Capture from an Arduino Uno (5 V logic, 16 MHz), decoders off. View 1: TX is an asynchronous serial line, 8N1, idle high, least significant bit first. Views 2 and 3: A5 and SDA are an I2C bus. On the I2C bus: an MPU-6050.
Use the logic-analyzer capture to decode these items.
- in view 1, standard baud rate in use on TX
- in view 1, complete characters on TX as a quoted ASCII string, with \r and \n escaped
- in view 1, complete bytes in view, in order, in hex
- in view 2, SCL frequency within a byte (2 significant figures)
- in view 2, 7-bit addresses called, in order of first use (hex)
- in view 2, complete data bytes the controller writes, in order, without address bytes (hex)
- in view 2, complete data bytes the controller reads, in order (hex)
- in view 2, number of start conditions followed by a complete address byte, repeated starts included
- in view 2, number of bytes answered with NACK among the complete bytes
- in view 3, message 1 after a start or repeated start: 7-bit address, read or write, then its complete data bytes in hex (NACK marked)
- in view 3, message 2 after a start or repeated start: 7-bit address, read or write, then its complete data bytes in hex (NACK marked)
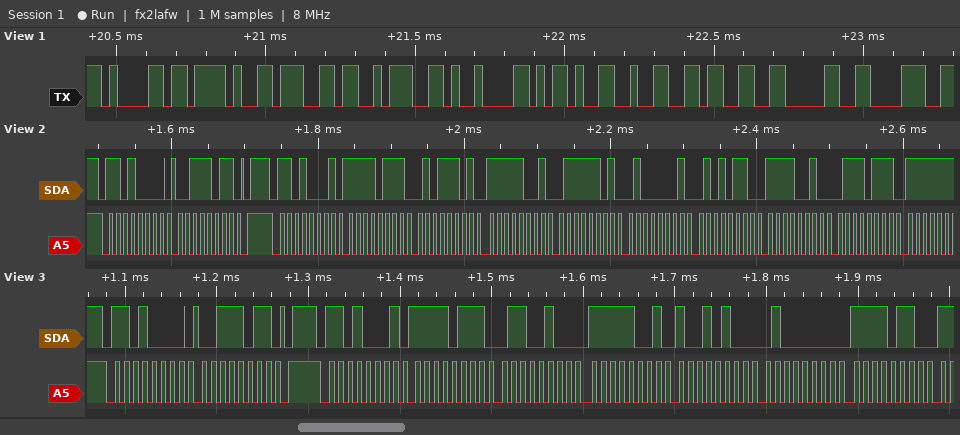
38400 baud
"a/g:\t-2308"
61 2F 67 3A 09 2D 32 33 30 38
100 kHz
0x68
3B
F7 5D F9 7D 41 56 F2 77
2
0
0x68 write: 3B
0x68 read: F7 64 F9 94 40 F6
